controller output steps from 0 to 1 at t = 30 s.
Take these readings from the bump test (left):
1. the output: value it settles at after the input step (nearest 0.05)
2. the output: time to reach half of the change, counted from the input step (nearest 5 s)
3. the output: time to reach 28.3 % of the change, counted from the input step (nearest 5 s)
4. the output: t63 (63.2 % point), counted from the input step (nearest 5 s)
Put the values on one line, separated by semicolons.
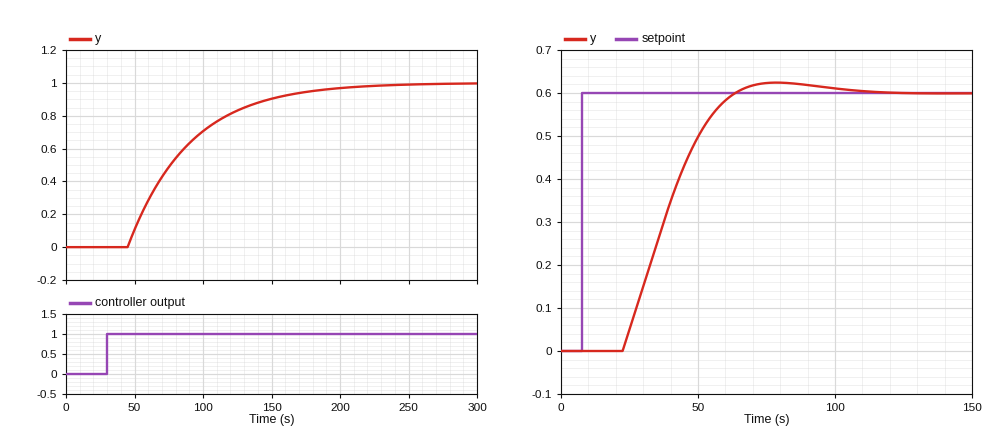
1.00; 45 s; 30 s; 60 s
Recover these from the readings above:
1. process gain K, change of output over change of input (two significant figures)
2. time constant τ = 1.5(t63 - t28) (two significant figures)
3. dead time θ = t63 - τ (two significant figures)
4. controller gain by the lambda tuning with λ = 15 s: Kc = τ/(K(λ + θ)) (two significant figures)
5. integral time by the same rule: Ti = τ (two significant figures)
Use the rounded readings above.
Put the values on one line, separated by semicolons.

1.0; 45 s; 15 s; 1.5; 45 s
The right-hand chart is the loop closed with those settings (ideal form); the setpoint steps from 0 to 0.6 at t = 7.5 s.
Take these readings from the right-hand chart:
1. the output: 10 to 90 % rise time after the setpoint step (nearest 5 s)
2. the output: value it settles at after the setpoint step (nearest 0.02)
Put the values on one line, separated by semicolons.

30 s; 0.60
